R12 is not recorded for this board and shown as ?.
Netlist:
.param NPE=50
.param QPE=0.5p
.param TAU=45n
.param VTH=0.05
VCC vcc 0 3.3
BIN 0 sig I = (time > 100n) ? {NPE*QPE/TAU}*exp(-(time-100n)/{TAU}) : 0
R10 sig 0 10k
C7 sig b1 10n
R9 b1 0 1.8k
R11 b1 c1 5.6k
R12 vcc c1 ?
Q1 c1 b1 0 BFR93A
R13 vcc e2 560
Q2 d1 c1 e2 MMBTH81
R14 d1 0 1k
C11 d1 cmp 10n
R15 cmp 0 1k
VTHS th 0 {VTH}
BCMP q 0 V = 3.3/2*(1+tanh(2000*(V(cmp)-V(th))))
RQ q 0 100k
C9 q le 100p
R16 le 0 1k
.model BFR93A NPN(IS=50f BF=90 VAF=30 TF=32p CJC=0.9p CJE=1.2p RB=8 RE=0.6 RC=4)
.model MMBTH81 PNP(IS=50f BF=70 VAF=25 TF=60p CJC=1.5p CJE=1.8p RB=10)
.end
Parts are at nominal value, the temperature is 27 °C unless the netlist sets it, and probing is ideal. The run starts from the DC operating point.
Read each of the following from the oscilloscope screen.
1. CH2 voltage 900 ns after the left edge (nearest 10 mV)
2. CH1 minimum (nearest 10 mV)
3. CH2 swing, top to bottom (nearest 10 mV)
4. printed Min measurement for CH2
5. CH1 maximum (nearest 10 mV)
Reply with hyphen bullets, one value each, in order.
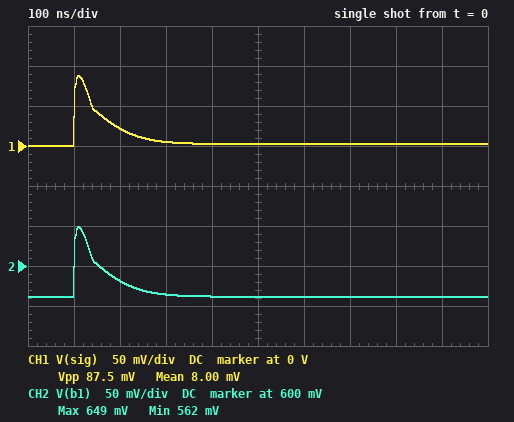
- 560 mV
- 0 V
- 90 mV
- 562 mV
- 90 mV
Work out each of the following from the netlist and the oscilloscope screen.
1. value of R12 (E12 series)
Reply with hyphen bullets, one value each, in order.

- 2.2 kΩ
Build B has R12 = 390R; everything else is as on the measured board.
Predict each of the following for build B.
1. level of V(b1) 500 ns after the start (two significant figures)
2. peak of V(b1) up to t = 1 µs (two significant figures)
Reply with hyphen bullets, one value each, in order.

- 620 mV
- 670 mV
